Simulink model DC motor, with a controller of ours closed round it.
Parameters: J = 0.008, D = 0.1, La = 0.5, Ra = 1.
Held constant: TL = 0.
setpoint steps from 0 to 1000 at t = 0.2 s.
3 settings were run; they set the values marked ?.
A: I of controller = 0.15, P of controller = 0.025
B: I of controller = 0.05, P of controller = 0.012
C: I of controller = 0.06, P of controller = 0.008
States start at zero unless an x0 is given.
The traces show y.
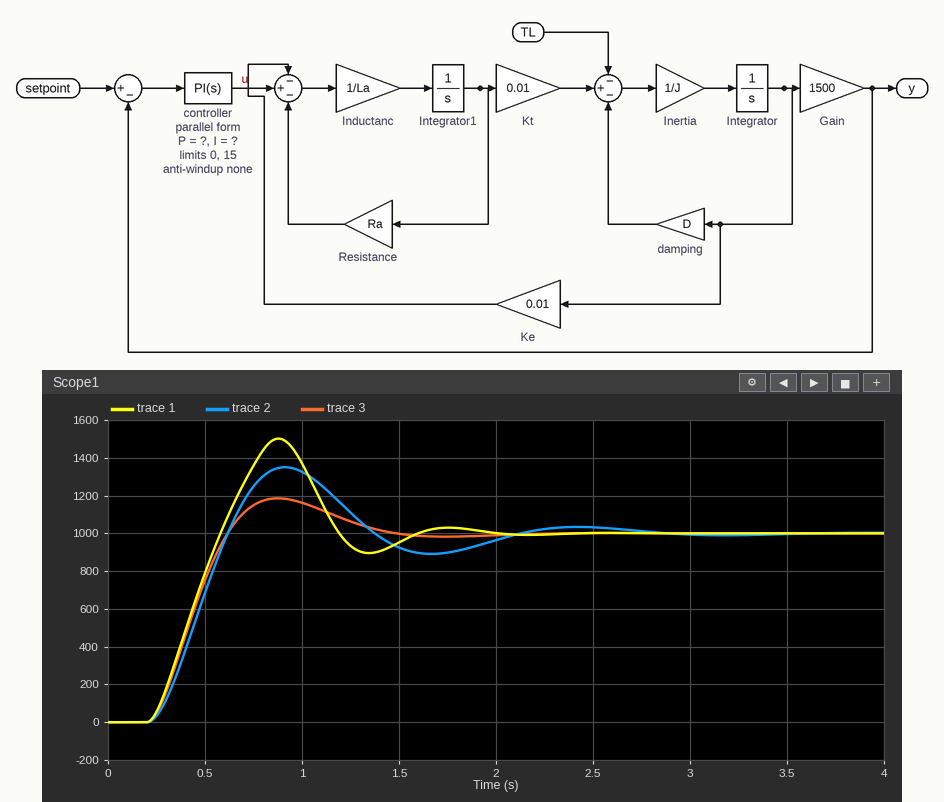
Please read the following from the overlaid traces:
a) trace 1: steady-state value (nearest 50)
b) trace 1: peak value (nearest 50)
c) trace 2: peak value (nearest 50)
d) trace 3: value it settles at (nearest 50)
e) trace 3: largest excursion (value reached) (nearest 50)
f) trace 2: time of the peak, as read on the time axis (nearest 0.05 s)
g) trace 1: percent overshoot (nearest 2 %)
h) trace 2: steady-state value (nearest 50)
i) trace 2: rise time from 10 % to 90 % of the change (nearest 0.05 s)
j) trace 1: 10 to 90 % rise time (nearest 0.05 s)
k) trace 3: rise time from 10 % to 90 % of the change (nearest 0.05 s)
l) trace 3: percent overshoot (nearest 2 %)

1000
1500
1350
1000
1200
0.90 s
50 %
1000
0.30 s
0.25 s
0.30 s
18 %
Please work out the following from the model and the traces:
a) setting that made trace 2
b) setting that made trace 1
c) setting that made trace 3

C
A
B
